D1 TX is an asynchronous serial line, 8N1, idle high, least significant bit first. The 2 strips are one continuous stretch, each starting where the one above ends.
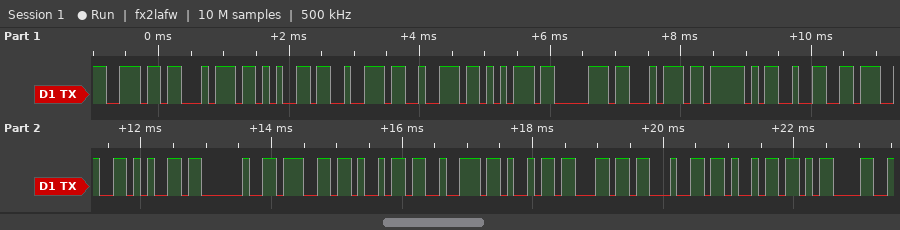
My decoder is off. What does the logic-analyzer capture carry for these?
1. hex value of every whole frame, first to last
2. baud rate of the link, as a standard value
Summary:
0x6E 0x74 0x65 0x72 0x72 0x75 0x70 0x74 0x5F 0x32 0x27 0x65 0x20 0x67 0x69 0x72 0x69 0x6C 0x64 0x69 0x0D
9600 baud
